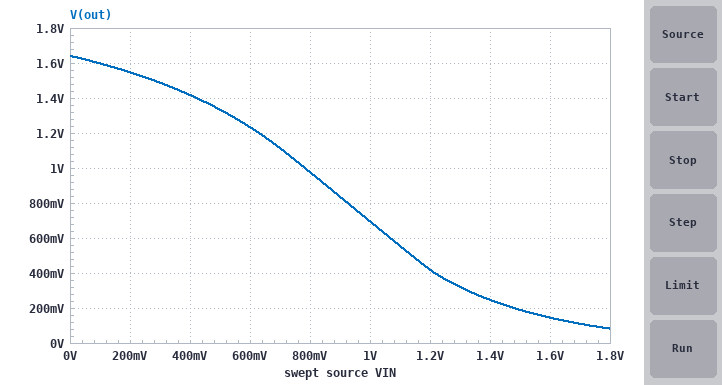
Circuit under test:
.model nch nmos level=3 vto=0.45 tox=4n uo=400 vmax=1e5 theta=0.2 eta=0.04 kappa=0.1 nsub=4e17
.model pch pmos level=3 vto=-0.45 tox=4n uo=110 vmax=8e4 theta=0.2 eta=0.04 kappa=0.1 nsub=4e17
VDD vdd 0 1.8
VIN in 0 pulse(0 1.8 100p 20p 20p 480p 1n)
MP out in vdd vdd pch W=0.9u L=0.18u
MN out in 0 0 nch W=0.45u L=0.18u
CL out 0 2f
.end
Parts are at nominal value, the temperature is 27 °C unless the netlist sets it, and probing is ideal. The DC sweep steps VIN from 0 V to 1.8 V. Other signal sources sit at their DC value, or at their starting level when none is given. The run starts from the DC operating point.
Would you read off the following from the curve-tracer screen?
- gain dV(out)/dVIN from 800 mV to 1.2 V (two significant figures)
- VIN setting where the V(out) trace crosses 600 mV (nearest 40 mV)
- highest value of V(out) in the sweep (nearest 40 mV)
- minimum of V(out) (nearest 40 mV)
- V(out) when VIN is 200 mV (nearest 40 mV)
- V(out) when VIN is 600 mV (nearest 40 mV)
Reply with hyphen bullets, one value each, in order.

- -1.4 V/V
- 1.08 V
- 1.64 V
- 80 mV
- 1.56 V
- 1.24 V
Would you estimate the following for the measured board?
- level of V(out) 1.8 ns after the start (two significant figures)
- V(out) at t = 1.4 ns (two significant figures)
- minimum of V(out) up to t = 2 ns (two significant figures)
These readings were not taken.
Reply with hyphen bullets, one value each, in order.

- 1.6 V
- 82 mV
- 75 mV
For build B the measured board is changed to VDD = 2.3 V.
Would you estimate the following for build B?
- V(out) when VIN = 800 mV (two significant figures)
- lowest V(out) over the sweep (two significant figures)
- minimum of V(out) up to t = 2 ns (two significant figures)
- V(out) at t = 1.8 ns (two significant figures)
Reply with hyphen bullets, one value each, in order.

- 1.6 V
- 340 mV
- 330 mV
- 2.1 V
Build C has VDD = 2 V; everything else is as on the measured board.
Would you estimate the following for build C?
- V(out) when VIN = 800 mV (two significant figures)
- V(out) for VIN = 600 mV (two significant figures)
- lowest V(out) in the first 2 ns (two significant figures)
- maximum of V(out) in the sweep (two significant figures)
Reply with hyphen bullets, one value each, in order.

- 1.2 V
- 1.4 V
- 160 mV
- 1.8 V
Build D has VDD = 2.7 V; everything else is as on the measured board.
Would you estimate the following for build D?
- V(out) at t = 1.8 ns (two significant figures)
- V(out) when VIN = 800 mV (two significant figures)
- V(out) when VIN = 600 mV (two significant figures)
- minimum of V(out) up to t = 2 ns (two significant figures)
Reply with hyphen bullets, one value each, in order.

- 2.4 V
- 2.0 V
- 2.1 V
- 740 mV
